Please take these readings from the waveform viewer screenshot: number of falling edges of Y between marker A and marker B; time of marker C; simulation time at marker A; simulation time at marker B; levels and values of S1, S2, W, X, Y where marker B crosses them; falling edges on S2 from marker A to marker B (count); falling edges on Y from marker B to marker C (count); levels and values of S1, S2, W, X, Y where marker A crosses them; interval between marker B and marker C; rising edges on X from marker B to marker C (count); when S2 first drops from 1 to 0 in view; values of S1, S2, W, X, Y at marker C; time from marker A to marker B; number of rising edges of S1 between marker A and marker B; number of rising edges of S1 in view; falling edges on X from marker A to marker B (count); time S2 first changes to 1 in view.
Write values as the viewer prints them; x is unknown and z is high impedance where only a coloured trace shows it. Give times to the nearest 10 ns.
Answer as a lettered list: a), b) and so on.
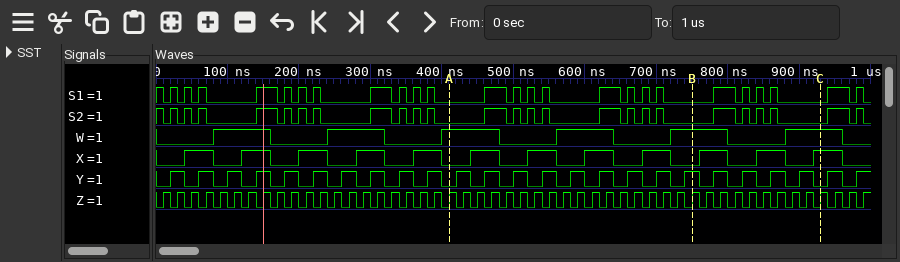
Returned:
a) 8
b) 930 ns
c) 410 ns
d) 750 ns
e) S1=0, S2=0, W=1, X=0, Y=1
f) 8
g) 5
h) S1=0, S2=0, W=1, X=0, Y=0
i) 180 ns
j) 3
k) 10 ns
l) S1=0, S2=0, W=1, X=1, Y=0
m) 340 ns
n) 8
o) 25
p) 4
q) 20 ns
